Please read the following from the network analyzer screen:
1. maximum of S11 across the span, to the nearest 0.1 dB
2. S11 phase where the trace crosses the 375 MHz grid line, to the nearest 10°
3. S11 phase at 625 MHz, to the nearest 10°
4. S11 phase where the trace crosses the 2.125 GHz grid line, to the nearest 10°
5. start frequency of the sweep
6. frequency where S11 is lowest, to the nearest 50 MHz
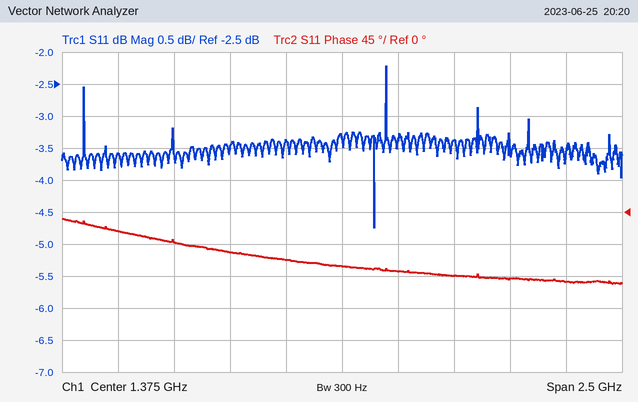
-2.2 dB
-30°
-40°
-90°
125 MHz
1.50 GHz
